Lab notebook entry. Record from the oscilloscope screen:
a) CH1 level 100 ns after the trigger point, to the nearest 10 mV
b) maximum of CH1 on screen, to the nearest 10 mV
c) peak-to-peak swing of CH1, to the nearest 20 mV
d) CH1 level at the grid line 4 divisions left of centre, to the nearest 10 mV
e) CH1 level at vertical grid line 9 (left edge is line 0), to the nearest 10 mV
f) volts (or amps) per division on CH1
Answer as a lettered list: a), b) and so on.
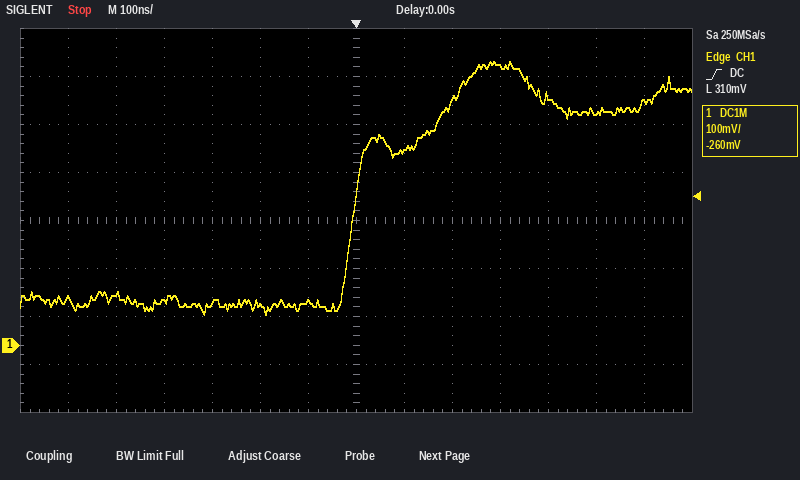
a) 400 mV
b) 590 mV
c) 520 mV
d) 90 mV
e) 510 mV
f) 100 mV
